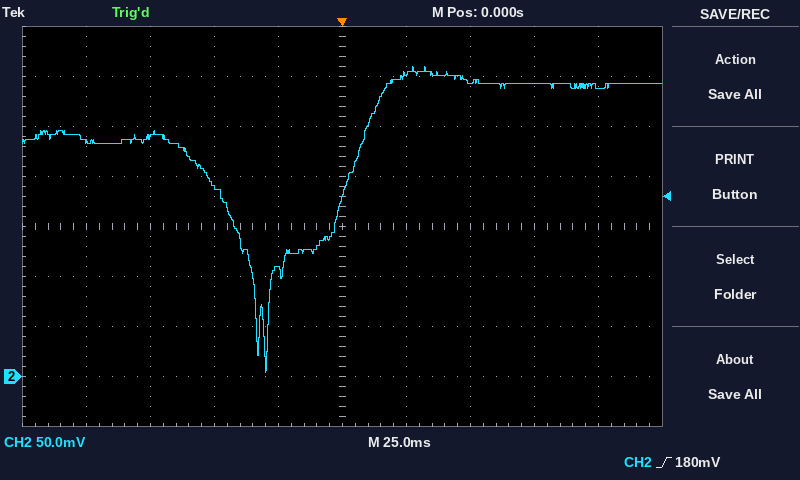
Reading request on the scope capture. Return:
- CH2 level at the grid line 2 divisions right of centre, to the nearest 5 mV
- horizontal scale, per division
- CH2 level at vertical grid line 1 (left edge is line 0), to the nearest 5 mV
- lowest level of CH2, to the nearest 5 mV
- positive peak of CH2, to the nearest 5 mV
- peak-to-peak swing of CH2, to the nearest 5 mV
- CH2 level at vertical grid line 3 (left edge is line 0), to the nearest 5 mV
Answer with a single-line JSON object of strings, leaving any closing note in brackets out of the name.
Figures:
{"CH2 level at the grid line 2 divisions right of centre, to the nearest 5 mV": "295 mV", "horizontal scale, per division": "25 ms", "CH2 level at vertical grid line 1 (left edge is line 0), to the nearest 5 mV": "235 mV", "lowest level of CH2, to the nearest 5 mV": "5 mV", "positive peak of CH2, to the nearest 5 mV": "310 mV", "peak-to-peak swing of CH2, to the nearest 5 mV": "305 mV", "CH2 level at vertical grid line 3 (left edge is line 0), to the nearest 5 mV": "190 mV"}
